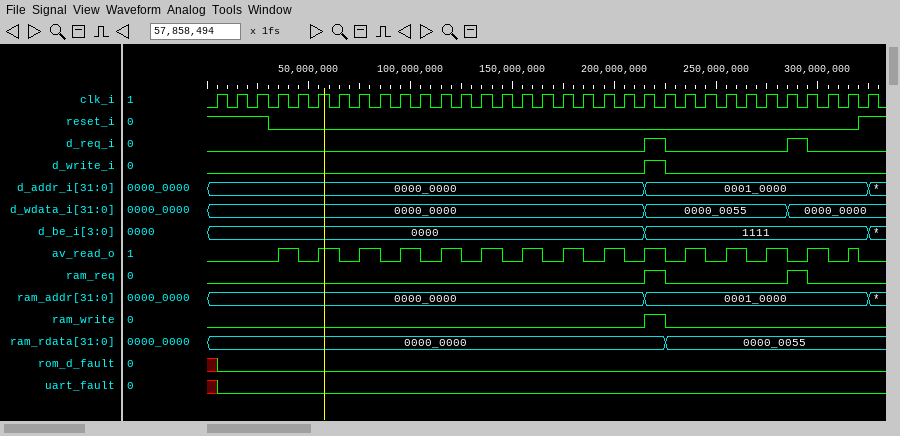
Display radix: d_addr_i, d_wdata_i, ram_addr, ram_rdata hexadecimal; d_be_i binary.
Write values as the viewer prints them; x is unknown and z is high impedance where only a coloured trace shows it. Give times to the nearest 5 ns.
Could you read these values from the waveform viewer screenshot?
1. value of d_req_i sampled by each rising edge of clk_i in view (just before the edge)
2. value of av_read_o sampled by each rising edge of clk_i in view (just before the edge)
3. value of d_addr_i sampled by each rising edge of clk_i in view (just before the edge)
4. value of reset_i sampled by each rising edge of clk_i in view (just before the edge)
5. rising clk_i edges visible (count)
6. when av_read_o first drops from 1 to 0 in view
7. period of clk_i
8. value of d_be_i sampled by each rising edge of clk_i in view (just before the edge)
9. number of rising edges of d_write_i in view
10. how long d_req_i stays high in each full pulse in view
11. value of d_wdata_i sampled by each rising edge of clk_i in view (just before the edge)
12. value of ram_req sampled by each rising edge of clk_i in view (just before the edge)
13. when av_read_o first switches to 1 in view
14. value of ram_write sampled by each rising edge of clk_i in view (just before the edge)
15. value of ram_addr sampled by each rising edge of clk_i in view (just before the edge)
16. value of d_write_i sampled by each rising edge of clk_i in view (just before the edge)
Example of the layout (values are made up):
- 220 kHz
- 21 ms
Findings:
- 0 0 0 0 0 0 0 0 0 0 0 0 0 0 0 0 0 0 0 0 0 0 1 0 0 0 0 0 0 1 0 0 0
- 0 0 0 0 1 0 1 0 1 0 1 0 1 0 1 0 1 0 1 0 1 0 1 0 1 0 1 0 1 0 1 0 0
- 0000_0000, 0000_0000, 0000_0000, 0000_0000, 0000_0000, 0000_0000, 0000_0000, 0000_0000, 0000_0000, 0000_0000, 0000_0000, 0000_0000, 0000_0000, 0000_0000, 0000_0000, 0000_0000, 0000_0000, 0000_0000, 0000_0000, 0000_0000, 0000_0000, 0000_0000, 0001_0000, 0001_0000, 0001_0000, 0001_0000, 0001_0000, 0001_0000, 0001_0000, 0001_0000, 0001_0000, 0001_0000, 0001_0000
- 1 1 1 0 0 0 0 0 0 0 0 0 0 0 0 0 0 0 0 0 0 0 0 0 0 0 0 0 0 0 0 0 1
- 33
- 45 ns
- 10 ns
- 0000, 0000, 0000, 0000, 0000, 0000, 0000, 0000, 0000, 0000, 0000, 0000, 0000, 0000, 0000, 0000, 0000, 0000, 0000, 0000, 0000, 0000, 1111, 1111, 1111, 1111, 1111, 1111, 1111, 1111, 1111, 1111, 1111
- 1
- 10 ns, 10 ns
- 0000_0000, 0000_0000, 0000_0000, 0000_0000, 0000_0000, 0000_0000, 0000_0000, 0000_0000, 0000_0000, 0000_0000, 0000_0000, 0000_0000, 0000_0000, 0000_0000, 0000_0000, 0000_0000, 0000_0000, 0000_0000, 0000_0000, 0000_0000, 0000_0000, 0000_0000, 0000_0055, 0000_0055, 0000_0055, 0000_0055, 0000_0055, 0000_0055, 0000_0055, 0000_0000, 0000_0000, 0000_0000, 0000_0000
- 0 0 0 0 0 0 0 0 0 0 0 0 0 0 0 0 0 0 0 0 0 0 1 0 0 0 0 0 0 1 0 0 0
- 35 ns
- 0 0 0 0 0 0 0 0 0 0 0 0 0 0 0 0 0 0 0 0 0 0 1 0 0 0 0 0 0 0 0 0 0
- 0000_0000, 0000_0000, 0000_0000, 0000_0000, 0000_0000, 0000_0000, 0000_0000, 0000_0000, 0000_0000, 0000_0000, 0000_0000, 0000_0000, 0000_0000, 0000_0000, 0000_0000, 0000_0000, 0000_0000, 0000_0000, 0000_0000, 0000_0000, 0000_0000, 0000_0000, 0001_0000, 0001_0000, 0001_0000, 0001_0000, 0001_0000, 0001_0000, 0001_0000, 0001_0000, 0001_0000, 0001_0000, 0001_0000
- 0 0 0 0 0 0 0 0 0 0 0 0 0 0 0 0 0 0 0 0 0 0 1 0 0 0 0 0 0 0 0 0 0
